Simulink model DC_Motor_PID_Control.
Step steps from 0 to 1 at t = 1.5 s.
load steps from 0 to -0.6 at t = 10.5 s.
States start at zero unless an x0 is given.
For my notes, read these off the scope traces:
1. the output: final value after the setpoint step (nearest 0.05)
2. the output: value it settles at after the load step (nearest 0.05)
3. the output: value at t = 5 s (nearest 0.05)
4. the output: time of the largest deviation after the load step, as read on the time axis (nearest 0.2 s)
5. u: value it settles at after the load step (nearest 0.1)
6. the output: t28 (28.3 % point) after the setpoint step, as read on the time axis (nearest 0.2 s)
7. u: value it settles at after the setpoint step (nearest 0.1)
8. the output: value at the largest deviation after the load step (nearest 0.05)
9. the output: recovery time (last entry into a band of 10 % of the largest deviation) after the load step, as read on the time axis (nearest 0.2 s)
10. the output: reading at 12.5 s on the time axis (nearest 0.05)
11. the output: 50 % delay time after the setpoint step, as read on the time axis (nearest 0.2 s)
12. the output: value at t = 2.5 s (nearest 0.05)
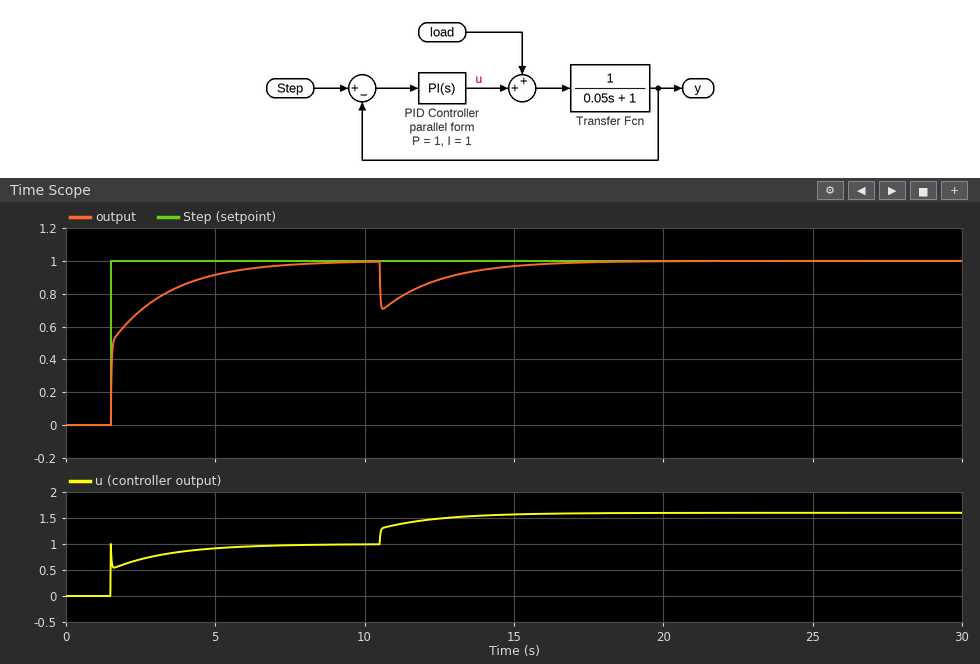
1.00
1.00
0.90
10.6 s
1.6
1.6 s
1.0
0.70
15.2 s
0.90
1.6 s
0.70
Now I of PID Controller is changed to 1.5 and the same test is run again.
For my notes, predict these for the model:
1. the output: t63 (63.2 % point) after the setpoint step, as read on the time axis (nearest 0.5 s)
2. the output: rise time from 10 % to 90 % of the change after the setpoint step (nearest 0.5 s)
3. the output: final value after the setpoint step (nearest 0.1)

2.0 s
2.0 s
1.0
